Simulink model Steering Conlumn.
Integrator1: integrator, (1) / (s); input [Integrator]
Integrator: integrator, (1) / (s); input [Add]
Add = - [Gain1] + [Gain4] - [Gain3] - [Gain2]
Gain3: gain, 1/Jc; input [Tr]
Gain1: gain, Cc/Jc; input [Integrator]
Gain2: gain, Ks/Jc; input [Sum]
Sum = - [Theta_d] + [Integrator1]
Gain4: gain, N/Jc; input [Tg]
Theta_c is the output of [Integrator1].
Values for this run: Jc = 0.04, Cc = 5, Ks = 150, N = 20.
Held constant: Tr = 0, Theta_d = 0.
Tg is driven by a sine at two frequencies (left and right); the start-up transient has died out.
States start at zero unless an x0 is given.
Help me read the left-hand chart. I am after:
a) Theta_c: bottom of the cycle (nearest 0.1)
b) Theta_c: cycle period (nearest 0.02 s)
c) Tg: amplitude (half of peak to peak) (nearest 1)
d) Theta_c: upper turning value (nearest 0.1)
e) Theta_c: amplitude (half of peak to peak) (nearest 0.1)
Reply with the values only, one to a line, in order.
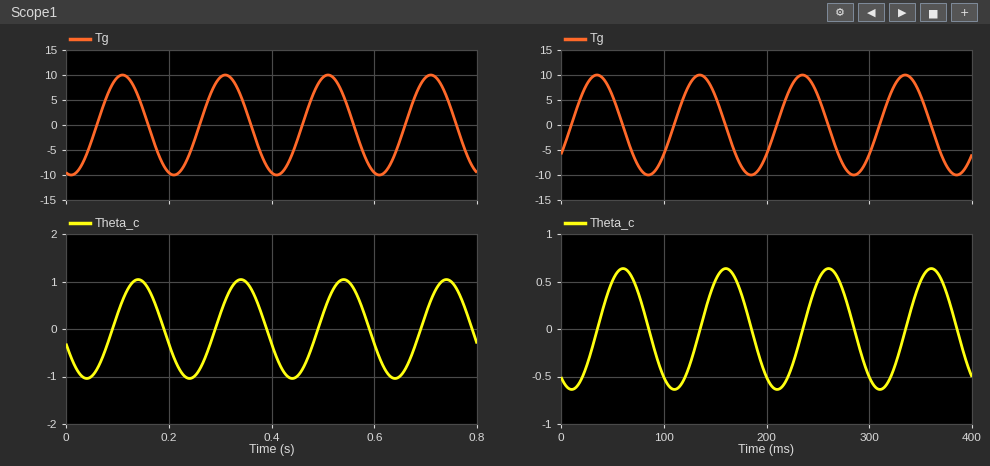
-1.0
0.20 s
10
1.0
1.0
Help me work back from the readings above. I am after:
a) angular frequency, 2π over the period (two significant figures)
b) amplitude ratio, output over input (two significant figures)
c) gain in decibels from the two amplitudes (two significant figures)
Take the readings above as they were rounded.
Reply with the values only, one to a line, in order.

31 rad/s
0.10
-20 dB
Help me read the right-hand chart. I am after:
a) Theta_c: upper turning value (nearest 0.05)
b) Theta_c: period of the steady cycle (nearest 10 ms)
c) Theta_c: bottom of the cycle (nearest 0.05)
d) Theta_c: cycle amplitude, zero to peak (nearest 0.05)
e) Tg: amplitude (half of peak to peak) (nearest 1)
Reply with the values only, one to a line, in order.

0.65
100 ms
-0.65
0.65
10
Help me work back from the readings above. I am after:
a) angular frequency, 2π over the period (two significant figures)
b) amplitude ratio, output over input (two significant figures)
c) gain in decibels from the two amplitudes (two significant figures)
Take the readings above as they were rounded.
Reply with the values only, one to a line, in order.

0.063 rad/ms
0.065
-24 dB
